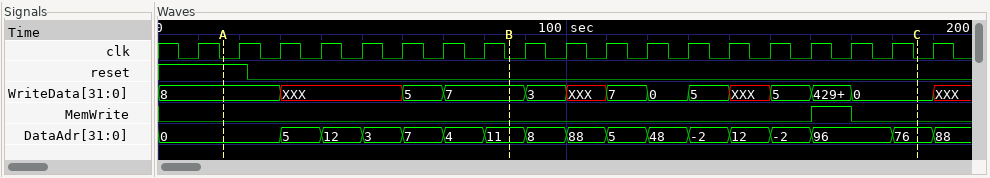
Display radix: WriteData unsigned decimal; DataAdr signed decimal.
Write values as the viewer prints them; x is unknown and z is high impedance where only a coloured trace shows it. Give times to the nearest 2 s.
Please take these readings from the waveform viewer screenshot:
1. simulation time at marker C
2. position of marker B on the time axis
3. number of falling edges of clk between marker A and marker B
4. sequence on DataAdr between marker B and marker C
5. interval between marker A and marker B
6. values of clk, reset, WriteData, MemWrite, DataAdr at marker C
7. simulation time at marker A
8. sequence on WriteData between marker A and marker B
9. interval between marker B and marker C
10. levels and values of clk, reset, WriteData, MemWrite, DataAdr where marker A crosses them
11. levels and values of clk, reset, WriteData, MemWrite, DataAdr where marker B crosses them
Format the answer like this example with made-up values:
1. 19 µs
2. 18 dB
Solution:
1. 186 s
2. 86 s
3. 7
4. 11, 8, 88, 5, 48, -2, 12, -2, 96, 76
5. 70 s
6. clk=0, reset=0, WriteData=0, MemWrite=0, DataAdr=76
7. 16 s
8. 8, XXX, 5, 7
9. 100 s
10. clk=0, reset=1, WriteData=8, MemWrite=0, DataAdr=0
11. clk=0, reset=0, WriteData=7, MemWrite=0, DataAdr=11
